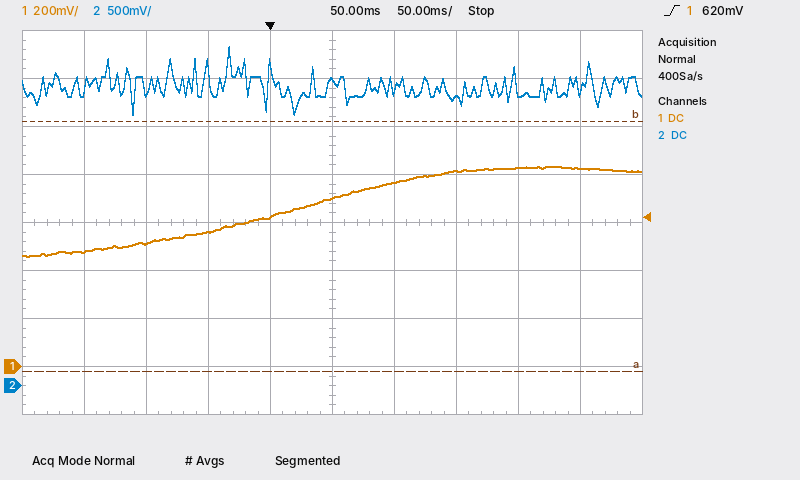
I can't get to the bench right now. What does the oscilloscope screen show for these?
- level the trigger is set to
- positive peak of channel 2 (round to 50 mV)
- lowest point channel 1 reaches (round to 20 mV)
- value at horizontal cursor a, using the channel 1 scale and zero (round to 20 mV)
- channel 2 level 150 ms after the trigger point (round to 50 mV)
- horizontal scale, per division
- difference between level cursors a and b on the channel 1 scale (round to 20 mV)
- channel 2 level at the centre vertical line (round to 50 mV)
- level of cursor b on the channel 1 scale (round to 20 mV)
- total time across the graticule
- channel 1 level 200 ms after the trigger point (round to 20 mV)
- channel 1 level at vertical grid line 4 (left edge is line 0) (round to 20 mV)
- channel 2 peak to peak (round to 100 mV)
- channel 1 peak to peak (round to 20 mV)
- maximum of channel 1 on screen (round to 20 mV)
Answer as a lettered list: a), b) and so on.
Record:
a) 620 mV
b) 3.55 V
c) 460 mV
d) -20 mV
e) 3.00 V
f) 50 ms
g) 1.04 V
h) 3.20 V
i) 1.02 V
j) 500 ms
k) 820 mV
l) 620 mV
m) 700 mV
n) 380 mV
o) 840 mV
